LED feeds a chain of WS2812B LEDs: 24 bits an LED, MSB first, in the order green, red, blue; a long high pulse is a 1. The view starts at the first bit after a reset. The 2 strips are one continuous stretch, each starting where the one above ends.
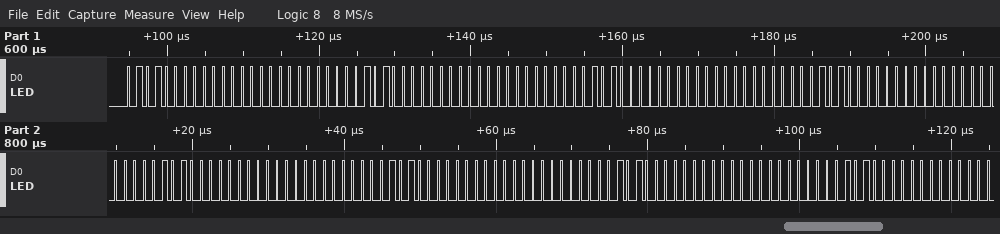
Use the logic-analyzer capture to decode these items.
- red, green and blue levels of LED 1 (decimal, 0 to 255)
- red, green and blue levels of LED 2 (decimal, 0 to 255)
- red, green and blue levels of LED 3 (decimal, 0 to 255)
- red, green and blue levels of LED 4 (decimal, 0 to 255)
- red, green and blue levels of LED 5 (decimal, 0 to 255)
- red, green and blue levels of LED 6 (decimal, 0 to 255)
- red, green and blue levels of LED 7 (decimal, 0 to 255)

0, 80, 0
0, 80, 0
0, 80, 0
0, 80, 0
0, 80, 0
0, 80, 0
0, 80, 0
